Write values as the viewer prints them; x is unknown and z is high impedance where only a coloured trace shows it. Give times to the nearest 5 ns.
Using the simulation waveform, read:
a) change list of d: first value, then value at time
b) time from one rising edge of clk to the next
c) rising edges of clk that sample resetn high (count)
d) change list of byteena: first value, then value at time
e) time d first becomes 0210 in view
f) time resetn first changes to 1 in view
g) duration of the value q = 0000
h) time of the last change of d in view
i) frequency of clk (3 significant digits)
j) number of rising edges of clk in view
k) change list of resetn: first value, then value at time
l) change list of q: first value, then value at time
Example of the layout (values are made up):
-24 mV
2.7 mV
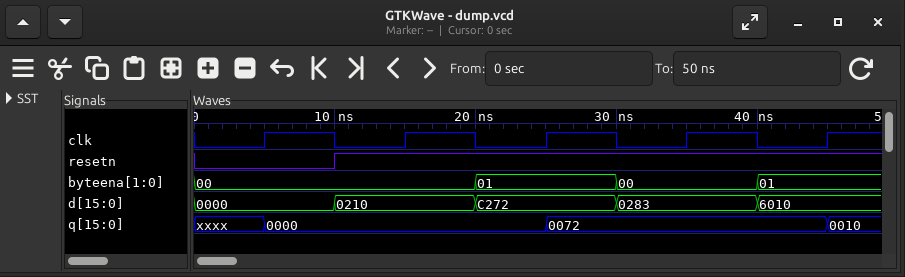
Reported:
0000, 0210 at 10 ns, C272 at 20 ns, 0283 at 30 ns, 6010 at 40 ns
10 ns
4
00, 01 at 20 ns, 00 at 30 ns, 01 at 40 ns
10 ns
10 ns
20 ns
40 ns
100 MHz
5
0, 1 at 10 ns
xxxx, 0000 at 5 ns, 0072 at 25 ns, 0010 at 45 ns
